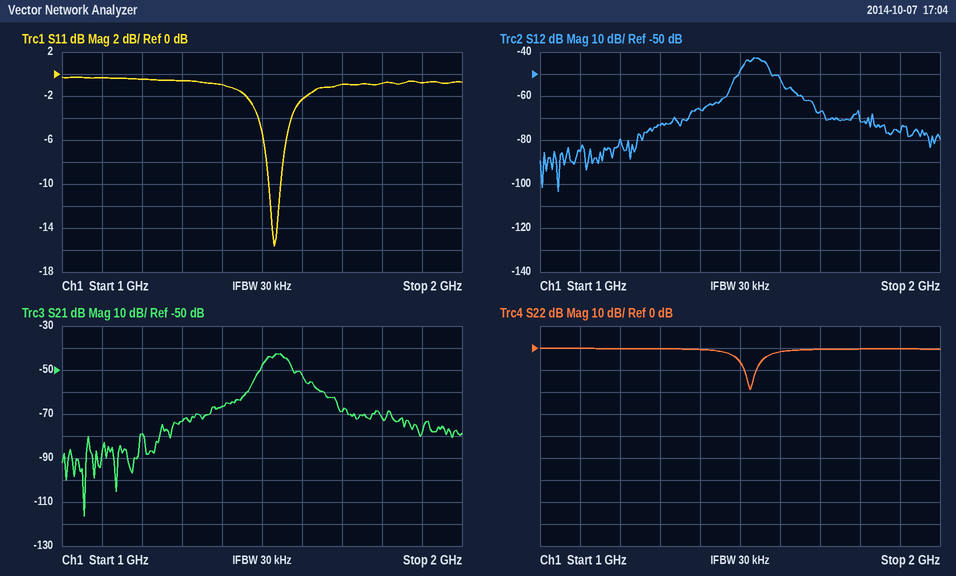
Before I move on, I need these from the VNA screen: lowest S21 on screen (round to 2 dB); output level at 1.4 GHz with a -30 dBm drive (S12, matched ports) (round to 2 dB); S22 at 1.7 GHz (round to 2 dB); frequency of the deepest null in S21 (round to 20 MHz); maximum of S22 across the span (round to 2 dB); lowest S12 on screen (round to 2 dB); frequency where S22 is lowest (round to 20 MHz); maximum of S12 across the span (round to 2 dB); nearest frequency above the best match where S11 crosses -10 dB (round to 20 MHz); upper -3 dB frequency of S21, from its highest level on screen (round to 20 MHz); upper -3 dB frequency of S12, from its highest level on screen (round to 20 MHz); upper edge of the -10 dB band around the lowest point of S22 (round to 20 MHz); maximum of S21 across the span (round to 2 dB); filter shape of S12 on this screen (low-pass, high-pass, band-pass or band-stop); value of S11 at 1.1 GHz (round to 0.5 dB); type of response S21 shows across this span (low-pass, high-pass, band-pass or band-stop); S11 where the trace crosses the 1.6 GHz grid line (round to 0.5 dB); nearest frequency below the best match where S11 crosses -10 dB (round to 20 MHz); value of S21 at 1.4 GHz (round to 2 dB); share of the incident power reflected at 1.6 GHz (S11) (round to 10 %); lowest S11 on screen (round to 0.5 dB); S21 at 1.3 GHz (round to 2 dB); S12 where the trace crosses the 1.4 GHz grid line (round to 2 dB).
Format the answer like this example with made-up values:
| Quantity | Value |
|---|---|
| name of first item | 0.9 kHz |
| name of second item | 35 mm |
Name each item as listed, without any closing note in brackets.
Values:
| Quantity | Value |
|---|---|
| lowest S21 on screen | -116 dB |
| output level at 1.4 GHz with a -30 dBm drive (S12, matched ports) | -96 dBm |
| S22 at 1.7 GHz | 0 dB |
| frequency of the deepest null in S21 | 1.06 GHz |
| maximum of S22 across the span | 0 dB |
| lowest S12 on screen | -104 dB |
| frequency where S22 is lowest | 1.52 GHz |
| maximum of S12 across the span | -42 dB |
| nearest frequency above the best match where S11 crosses -10 dB | 1.54 GHz |
| upper -3 dB frequency of S21, from its highest level on screen | 1.56 GHz |
| upper -3 dB frequency of S12, from its highest level on screen | 1.56 GHz |
| upper edge of the -10 dB band around the lowest point of S22 | 1.54 GHz |
| maximum of S21 across the span | -42 dB |
| filter shape of S12 on this screen | band-pass |
| value of S11 at 1.1 GHz | -0.5 dB |
| type of response S21 shows across this span | band-pass |
| S11 where the trace crosses the 1.6 GHz grid line | -2.5 dB |
| nearest frequency below the best match where S11 crosses -10 dB | 1.52 GHz |
| value of S21 at 1.4 GHz | -66 dB |
| share of the incident power reflected at 1.6 GHz (S11) | 60 % |
| lowest S11 on screen | -15.5 dB |
| S21 at 1.3 GHz | -74 dB |
| S12 where the trace crosses the 1.4 GHz grid line | -66 dB |
